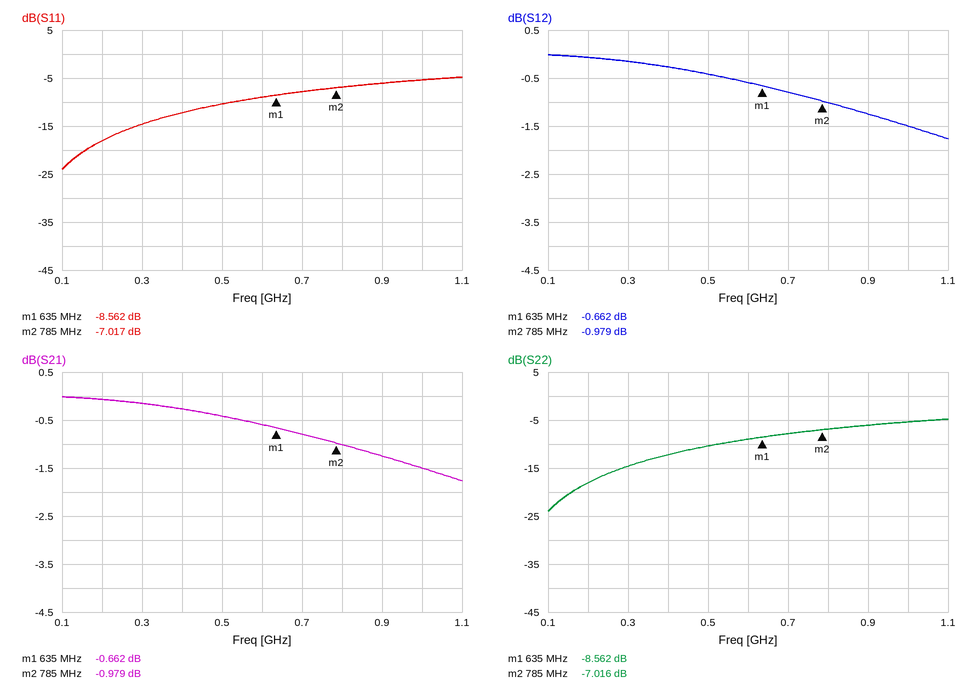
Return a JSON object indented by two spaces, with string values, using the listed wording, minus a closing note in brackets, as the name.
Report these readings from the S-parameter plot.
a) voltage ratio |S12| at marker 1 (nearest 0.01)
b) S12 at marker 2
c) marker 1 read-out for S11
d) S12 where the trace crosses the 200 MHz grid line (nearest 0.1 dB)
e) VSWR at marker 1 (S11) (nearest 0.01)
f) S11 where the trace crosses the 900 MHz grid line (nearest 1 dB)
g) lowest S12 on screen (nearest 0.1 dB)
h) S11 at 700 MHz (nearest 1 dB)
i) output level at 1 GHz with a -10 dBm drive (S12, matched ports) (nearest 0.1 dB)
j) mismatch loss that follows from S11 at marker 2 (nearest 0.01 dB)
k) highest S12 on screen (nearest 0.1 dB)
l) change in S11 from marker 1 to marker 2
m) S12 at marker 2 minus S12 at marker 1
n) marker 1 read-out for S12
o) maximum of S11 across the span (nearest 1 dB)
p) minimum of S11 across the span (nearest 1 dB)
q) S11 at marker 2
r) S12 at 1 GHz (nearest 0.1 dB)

{
  "voltage ratio |S12| at marker 1": "0.93",
  "S12 at marker 2": "-0.979 dB",
  "marker 1 read-out for S11": "-8.562 dB",
  "S12 where the trace crosses the 200 MHz grid line": "-0.1 dB",
  "VSWR at marker 1 (S11)": "2.19",
  "S11 where the trace crosses the 900 MHz grid line": "-6 dB",
  "lowest S12 on screen": "-1.8 dB",
  "S11 at 700 MHz": "-8 dB",
  "output level at 1 GHz with a -10 dBm drive (S12, matched ports)": "-11.5 dBm",
  "mismatch loss that follows from S11 at marker 2": "0.96 dB",
  "highest S12 on screen": "0.0 dB",
  "change in S11 from marker 1 to marker 2": "1.545 dB",
  "S12 at marker 2 minus S12 at marker 1": "-0.317 dB",
  "marker 1 read-out for S12": "-0.662 dB",
  "maximum of S11 across the span": "-5 dB",
  "minimum of S11 across the span": "-24 dB",
  "S11 at marker 2": "-7.017 dB",
  "S12 at 1 GHz": "-1.5 dB"
}
